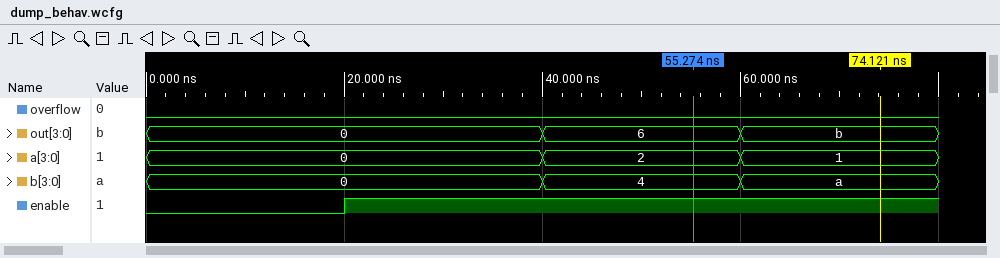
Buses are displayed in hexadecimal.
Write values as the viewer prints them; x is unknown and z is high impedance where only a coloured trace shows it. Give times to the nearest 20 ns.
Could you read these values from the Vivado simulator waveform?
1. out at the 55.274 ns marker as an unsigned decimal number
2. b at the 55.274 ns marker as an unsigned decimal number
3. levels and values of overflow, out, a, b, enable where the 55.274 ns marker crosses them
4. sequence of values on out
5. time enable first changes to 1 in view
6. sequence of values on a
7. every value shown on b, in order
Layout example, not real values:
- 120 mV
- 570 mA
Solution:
- 6
- 4
- overflow=0, out=6, a=2, b=4, enable=1
- 0, 6, b
- 20 ns
- 0, 2, 1
- 0, 4, a
